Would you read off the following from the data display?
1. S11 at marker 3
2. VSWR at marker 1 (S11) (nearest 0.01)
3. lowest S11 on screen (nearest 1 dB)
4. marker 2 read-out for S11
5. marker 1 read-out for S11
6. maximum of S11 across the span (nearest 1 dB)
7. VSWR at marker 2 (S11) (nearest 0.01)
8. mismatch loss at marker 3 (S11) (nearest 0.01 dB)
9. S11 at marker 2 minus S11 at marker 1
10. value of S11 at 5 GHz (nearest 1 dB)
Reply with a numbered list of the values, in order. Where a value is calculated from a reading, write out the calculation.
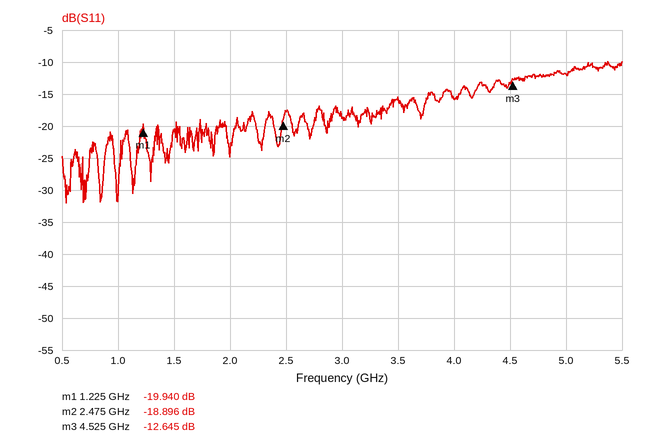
1. -12.645 dB
2. (1 + 0.1007)/(1 − 0.1007) ≈ 1.22
3. -32 dB
4. -18.896 dB
5. -19.940 dB
6. -10 dB
7. (1 + 0.1136)/(1 − 0.1136) ≈ 1.26
8. −10 log10(1 − 10^(-12.645/10)) ≈ 0.24 dB
9. -18.896 − (-19.94) = 1.044 dB
10. -12 dB
